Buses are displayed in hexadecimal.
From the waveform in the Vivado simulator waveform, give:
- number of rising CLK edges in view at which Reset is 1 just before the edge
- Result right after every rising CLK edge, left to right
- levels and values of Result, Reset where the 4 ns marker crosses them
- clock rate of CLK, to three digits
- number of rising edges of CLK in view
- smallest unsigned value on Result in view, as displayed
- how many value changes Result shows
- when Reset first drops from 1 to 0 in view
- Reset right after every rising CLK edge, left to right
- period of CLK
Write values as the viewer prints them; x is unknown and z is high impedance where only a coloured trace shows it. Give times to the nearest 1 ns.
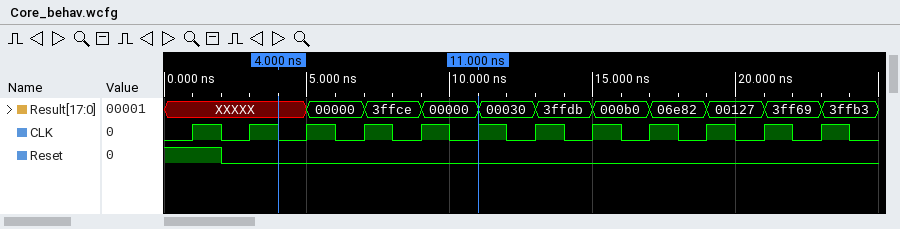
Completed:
1
XXXXX, XXXXX, 00000, 3ffce, 00000, 00030, 3ffdb, 000b0, 06e82, 00127, 3ff69, 3ffb3
Result=XXXXX, Reset=0
500 MHz
12
00000
10
2 ns
1 0 0 0 0 0 0 0 0 0 0 0
2 ns
